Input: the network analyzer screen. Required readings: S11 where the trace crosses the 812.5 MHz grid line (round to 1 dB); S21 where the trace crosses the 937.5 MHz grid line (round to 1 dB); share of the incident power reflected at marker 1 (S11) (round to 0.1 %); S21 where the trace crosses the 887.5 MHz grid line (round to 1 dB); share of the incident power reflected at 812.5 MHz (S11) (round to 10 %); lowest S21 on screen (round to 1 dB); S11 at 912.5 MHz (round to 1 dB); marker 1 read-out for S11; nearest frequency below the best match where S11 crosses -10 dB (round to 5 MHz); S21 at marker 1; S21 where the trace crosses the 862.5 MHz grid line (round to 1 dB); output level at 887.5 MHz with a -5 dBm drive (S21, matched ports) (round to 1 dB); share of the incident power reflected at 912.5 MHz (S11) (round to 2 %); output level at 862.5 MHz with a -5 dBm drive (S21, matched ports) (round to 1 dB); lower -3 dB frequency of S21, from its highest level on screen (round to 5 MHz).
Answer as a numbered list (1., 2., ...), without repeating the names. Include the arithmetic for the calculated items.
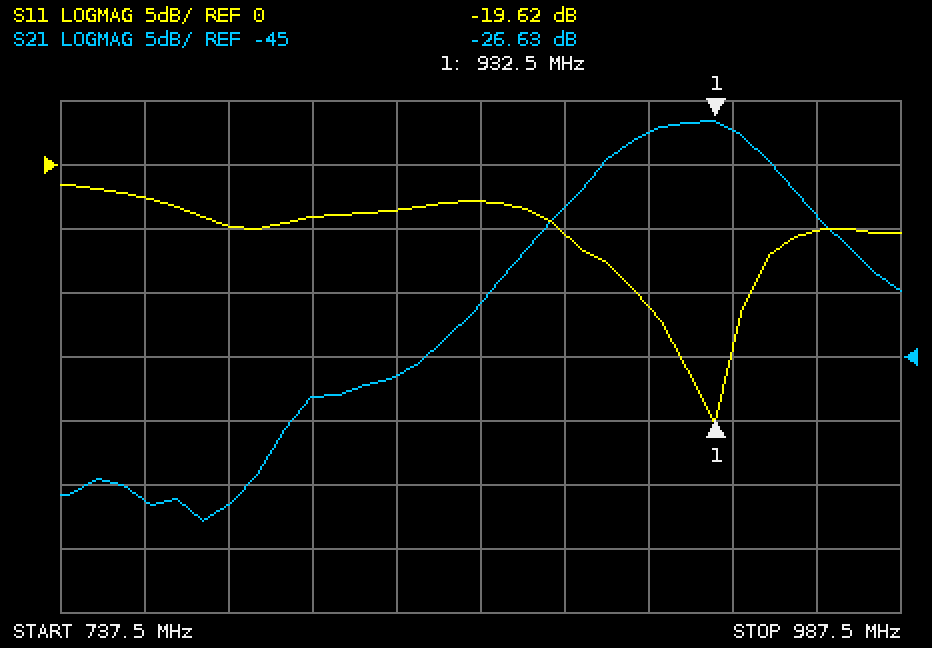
1. -4 dB
2. -27 dB
3. 10^(-19.62/10) ≈ 1.1 %
4. -33 dB
5. 10^(-4/10) ≈ 40 %
6. -58 dB
7. -11 dB
8. -19.62 dB
9. 910 MHz
10. -26.63 dB
11. -41 dB
12. -5 dBm + (-33 dB) = -38 dBm
13. 10^(-11/10) ≈ 8 %
14. -5 dBm + (-41 dB) = -46 dBm
15. 900 MHz
